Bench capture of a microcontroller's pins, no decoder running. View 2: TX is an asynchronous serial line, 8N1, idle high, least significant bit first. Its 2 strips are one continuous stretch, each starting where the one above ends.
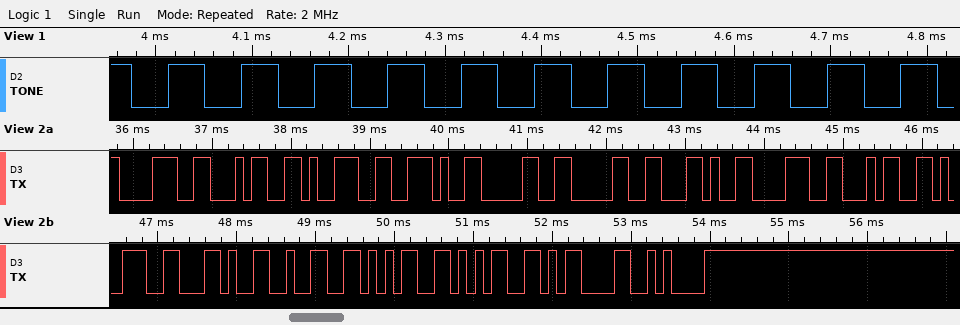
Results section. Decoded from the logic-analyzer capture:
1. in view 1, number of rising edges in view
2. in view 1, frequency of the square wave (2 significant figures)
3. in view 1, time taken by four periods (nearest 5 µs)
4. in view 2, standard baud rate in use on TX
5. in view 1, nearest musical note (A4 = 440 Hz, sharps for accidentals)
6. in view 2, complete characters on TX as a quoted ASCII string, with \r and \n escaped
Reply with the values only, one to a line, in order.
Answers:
11
13 kHz
305 µs
9600 baud
G#9
"849.00,849,255\r\n"
